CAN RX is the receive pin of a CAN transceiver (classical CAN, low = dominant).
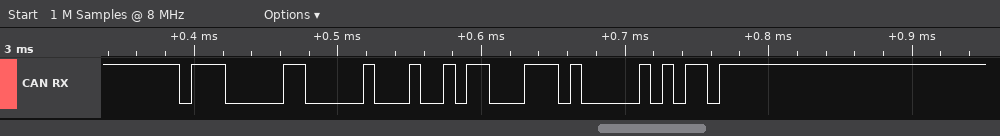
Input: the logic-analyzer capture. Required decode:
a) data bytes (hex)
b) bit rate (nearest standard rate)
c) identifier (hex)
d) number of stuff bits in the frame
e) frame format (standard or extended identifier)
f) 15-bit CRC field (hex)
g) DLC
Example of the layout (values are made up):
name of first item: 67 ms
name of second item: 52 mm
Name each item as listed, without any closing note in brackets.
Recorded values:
data bytes: 2C
bit rate: 125 kbit/s
identifier: 0x704
number of stuff bits in the frame: 3
frame format: standard
15-bit CRC field: 0x3A05
DLC: 1
